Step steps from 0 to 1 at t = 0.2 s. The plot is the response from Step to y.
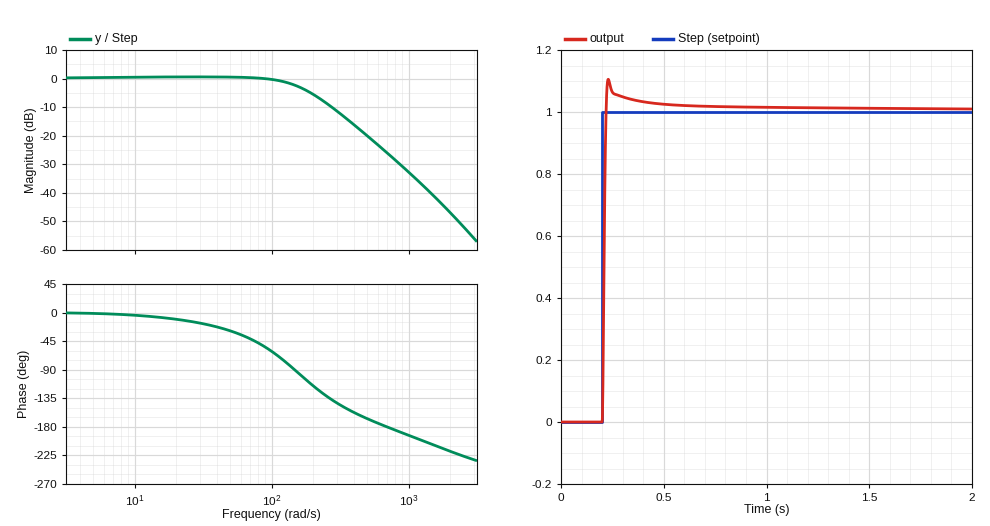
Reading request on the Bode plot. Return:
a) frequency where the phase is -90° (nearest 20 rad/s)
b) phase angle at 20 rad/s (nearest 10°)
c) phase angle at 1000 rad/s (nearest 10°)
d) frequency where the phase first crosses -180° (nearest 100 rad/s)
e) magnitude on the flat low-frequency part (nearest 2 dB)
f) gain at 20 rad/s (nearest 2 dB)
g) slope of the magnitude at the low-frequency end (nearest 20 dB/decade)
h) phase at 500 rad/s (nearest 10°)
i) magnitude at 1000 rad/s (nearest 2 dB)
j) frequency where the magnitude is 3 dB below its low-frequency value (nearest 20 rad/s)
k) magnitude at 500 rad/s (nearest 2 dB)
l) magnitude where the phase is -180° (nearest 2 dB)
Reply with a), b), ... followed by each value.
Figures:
a) 140 rad/s
b) -10°
c) -190°
d) 700 rad/s
e) 0 dB
f) 0 dB
g) 0 dB/decade
h) -170°
i) -32 dB
j) 160 rad/s
k) -20 dB
l) -26 dB
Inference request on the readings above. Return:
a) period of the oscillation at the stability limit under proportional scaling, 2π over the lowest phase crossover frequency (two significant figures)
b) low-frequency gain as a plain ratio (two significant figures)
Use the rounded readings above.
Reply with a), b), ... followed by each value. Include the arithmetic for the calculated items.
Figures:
a) 2π / 700 = 0.0090 s
b) 10^(0 / 20) = 1.0
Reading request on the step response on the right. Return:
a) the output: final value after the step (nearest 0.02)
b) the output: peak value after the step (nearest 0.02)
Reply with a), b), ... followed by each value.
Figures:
a) 1.00
b) 1.10
